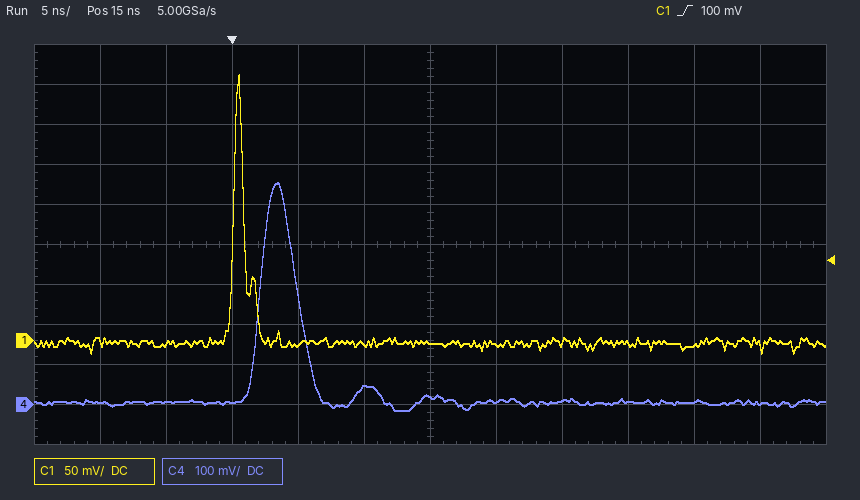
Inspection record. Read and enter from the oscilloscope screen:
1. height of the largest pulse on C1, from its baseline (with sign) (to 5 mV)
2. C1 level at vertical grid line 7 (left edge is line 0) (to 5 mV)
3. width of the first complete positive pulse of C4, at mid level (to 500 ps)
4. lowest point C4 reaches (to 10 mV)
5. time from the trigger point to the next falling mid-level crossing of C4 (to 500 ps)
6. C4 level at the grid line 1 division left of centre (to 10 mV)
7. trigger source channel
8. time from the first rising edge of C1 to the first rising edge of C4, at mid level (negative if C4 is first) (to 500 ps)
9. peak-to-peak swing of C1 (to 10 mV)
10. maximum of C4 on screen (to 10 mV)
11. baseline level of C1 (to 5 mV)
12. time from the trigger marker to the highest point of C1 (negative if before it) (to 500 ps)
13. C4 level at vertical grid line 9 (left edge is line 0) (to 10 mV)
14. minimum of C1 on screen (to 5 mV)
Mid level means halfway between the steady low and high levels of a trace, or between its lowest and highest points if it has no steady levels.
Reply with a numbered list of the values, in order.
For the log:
1. +335 mV
2. -5 mV
3. 3.0 ns
4. -20 mV
5. 5.0 ns
6. 40 mV
7. C1
8. +2.0 ns
9. 350 mV
10. 560 mV
11. -5 mV
12. +500 ps
13. 10 mV
14. -15 mV
